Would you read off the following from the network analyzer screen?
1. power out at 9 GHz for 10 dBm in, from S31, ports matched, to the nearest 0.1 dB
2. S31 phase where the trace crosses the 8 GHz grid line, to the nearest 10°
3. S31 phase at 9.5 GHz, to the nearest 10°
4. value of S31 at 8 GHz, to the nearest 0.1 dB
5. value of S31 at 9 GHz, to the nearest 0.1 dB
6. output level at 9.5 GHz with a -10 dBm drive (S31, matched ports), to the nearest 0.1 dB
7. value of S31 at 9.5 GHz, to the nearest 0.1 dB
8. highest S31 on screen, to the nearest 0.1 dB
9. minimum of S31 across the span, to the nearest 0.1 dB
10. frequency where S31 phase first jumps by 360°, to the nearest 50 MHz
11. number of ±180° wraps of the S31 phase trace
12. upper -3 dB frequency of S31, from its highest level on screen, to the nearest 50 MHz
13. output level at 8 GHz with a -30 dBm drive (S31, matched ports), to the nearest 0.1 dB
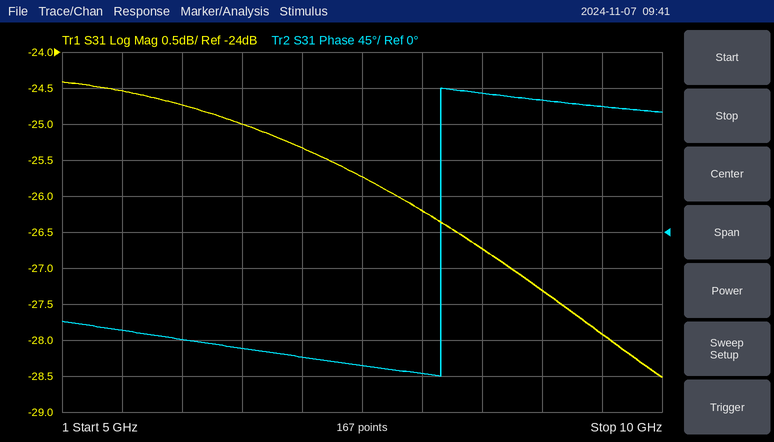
-17.3 dBm
-180°
160°
-26.2 dB
-27.3 dB
-37.9 dBm
-27.9 dB
-24.4 dB
-28.5 dB
8.15 GHz
1
9.10 GHz
-56.2 dBm
